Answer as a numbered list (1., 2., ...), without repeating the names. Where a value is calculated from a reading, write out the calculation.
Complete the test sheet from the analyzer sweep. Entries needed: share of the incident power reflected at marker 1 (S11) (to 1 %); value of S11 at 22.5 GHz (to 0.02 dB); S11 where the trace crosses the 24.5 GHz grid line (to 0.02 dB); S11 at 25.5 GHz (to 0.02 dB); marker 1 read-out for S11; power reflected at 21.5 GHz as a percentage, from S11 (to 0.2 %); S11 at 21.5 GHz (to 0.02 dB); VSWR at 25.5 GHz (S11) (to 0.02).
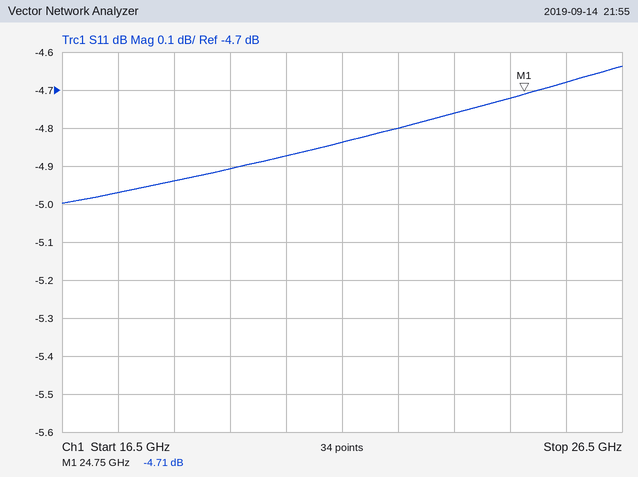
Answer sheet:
1. 10^(-4.71/10) ≈ 34 %
2. -4.80 dB
3. -4.72 dB
4. -4.68 dB
5. -4.71 dB
6. 10^(-4.84/10) ≈ 32.8 %
7. -4.84 dB
8. |Γ| = 10^(-4.68/20) = 0.5834; VSWR = (1 + 0.5834)/(1 − 0.5834) ≈ 3.80
